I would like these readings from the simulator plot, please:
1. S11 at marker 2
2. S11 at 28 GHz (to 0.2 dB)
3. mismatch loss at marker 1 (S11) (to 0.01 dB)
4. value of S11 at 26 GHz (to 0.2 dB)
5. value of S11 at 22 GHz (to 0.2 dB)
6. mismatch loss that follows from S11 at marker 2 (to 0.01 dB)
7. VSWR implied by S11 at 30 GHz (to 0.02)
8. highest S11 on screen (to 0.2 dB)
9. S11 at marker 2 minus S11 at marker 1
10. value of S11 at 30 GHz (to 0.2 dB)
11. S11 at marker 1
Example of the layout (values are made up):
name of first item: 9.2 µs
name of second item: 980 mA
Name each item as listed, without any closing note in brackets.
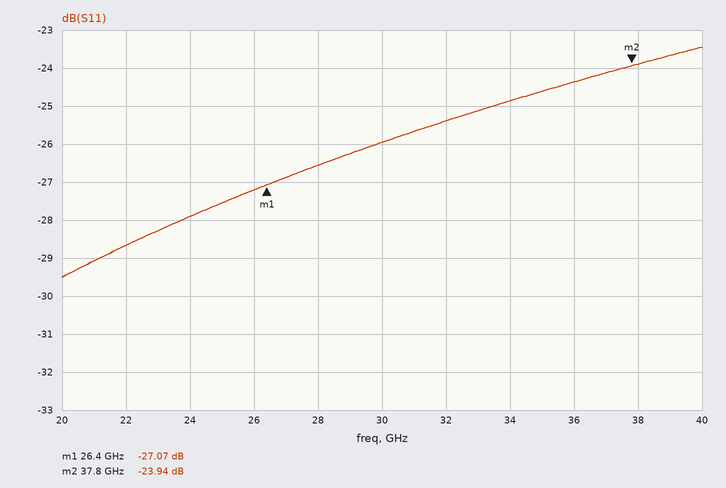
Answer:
S11 at marker 2: -23.94 dB
S11 at 28 GHz: -26.6 dB
mismatch loss at marker 1 (S11): 0.01 dB
value of S11 at 26 GHz: -27.2 dB
value of S11 at 22 GHz: -28.6 dB
mismatch loss that follows from S11 at marker 2: 0.02 dB
VSWR implied by S11 at 30 GHz: 1.10
highest S11 on screen: -23.4 dB
S11 at marker 2 minus S11 at marker 1: 3.13 dB
value of S11 at 30 GHz: -26.0 dB
S11 at marker 1: -27.07 dB
